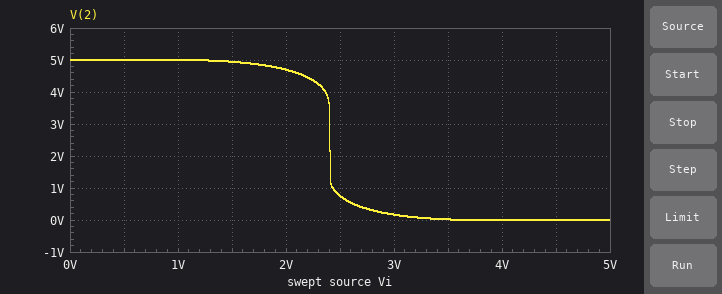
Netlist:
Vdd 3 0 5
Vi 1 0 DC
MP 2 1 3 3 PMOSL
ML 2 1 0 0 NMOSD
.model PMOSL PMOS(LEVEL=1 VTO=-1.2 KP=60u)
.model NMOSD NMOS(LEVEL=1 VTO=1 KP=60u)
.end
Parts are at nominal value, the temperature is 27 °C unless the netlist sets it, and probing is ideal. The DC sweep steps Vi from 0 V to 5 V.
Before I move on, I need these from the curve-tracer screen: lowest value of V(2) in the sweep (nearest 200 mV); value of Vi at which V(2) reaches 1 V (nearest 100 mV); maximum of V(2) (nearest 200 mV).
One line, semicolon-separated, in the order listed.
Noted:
0 V; 2.4 V; 5.0 V
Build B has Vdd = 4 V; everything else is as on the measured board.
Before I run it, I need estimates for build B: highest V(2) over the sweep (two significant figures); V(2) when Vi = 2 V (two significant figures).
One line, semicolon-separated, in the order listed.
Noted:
4.0 V; 400 mV
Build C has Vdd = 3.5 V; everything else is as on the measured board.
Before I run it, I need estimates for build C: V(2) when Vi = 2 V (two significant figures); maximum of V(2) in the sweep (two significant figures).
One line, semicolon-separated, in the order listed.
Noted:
46 mV; 3.5 V
